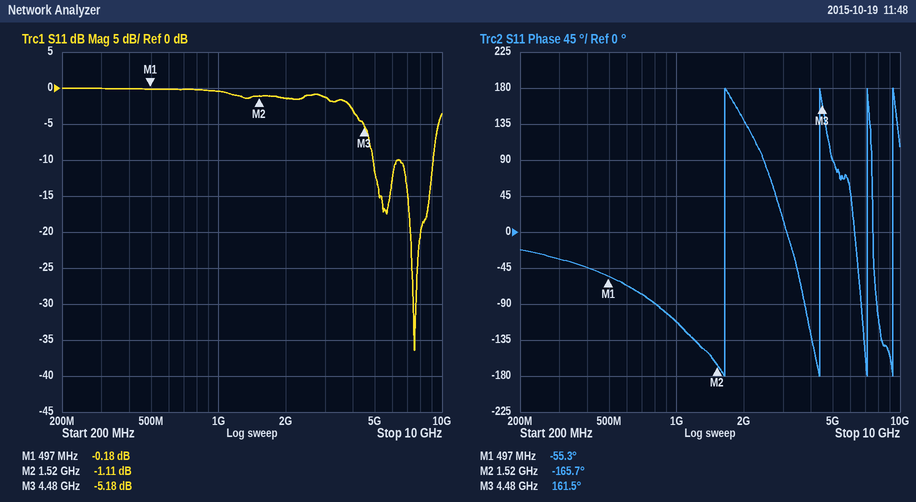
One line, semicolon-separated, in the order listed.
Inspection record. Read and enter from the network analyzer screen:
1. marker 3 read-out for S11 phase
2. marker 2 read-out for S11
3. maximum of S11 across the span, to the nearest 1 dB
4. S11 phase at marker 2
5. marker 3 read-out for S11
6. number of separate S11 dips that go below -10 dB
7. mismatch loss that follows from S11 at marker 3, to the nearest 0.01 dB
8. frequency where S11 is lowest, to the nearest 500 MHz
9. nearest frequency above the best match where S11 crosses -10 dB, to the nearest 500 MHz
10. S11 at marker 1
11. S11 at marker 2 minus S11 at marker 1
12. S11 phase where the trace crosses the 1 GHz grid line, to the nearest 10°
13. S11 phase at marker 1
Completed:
161.5°; -1.11 dB; 0 dB; -165.7°; -5.18 dB; 2; 1.57 dB; 7.5 GHz; 9.0 GHz; -0.18 dB; -0.93 dB; -110°; -55.3°
